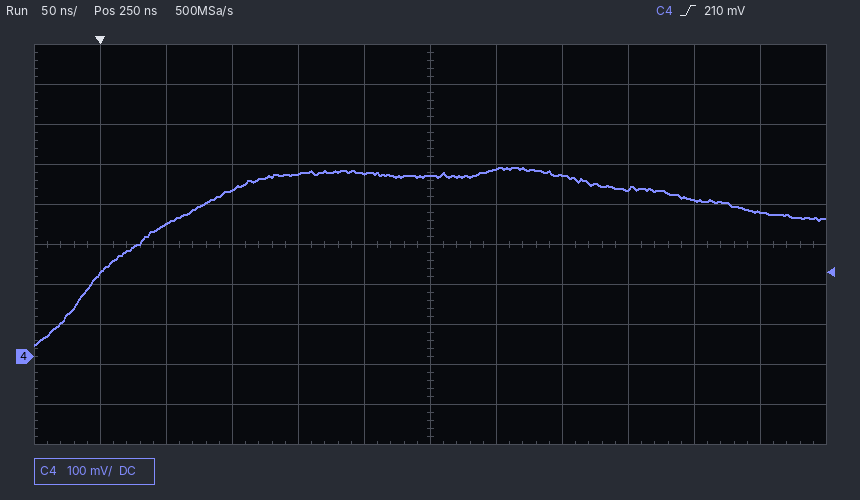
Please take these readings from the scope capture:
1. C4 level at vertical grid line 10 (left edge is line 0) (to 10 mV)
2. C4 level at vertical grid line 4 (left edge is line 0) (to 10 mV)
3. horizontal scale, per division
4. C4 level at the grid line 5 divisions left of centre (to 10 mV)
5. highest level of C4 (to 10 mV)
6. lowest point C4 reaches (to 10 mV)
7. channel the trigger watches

390 mV
460 mV
50 ns
210 mV
470 mV
30 mV
C4
